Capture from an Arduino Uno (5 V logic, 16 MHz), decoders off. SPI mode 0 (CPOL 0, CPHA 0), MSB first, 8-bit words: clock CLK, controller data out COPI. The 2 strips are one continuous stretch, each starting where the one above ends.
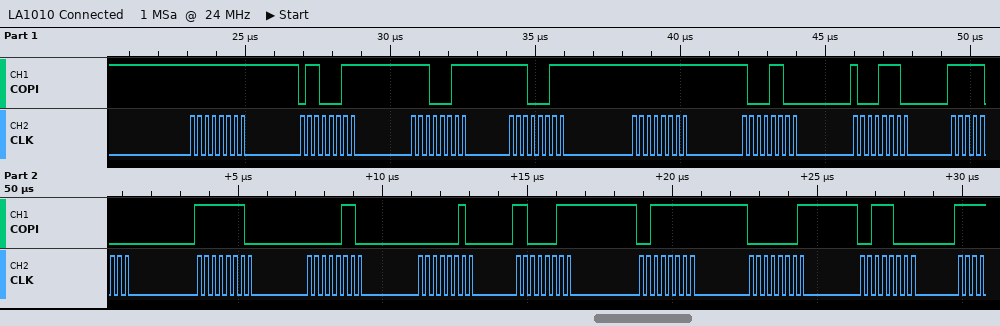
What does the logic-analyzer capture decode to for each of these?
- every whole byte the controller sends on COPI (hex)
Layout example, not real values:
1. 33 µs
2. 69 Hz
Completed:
1. FF 63 E3 E3 FF 8C 8E F8 FE 06 02 C3 3F 01 38
